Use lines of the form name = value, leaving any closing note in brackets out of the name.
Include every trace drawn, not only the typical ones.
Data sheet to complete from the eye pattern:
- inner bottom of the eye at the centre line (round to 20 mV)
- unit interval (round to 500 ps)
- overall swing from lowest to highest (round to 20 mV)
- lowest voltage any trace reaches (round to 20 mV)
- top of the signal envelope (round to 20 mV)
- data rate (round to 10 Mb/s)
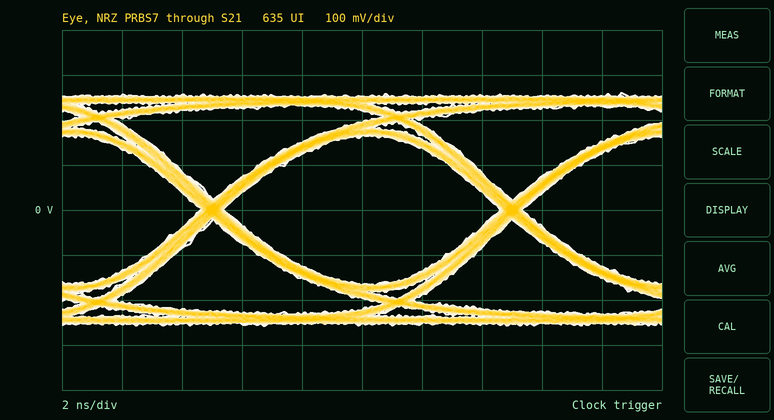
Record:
inner bottom of the eye at the centre line = -160 mV
unit interval = 10.0 ns
overall swing from lowest to highest = 520 mV
lowest voltage any trace reaches = -260 mV
top of the signal envelope = 260 mV
data rate = 100 Mb/s
